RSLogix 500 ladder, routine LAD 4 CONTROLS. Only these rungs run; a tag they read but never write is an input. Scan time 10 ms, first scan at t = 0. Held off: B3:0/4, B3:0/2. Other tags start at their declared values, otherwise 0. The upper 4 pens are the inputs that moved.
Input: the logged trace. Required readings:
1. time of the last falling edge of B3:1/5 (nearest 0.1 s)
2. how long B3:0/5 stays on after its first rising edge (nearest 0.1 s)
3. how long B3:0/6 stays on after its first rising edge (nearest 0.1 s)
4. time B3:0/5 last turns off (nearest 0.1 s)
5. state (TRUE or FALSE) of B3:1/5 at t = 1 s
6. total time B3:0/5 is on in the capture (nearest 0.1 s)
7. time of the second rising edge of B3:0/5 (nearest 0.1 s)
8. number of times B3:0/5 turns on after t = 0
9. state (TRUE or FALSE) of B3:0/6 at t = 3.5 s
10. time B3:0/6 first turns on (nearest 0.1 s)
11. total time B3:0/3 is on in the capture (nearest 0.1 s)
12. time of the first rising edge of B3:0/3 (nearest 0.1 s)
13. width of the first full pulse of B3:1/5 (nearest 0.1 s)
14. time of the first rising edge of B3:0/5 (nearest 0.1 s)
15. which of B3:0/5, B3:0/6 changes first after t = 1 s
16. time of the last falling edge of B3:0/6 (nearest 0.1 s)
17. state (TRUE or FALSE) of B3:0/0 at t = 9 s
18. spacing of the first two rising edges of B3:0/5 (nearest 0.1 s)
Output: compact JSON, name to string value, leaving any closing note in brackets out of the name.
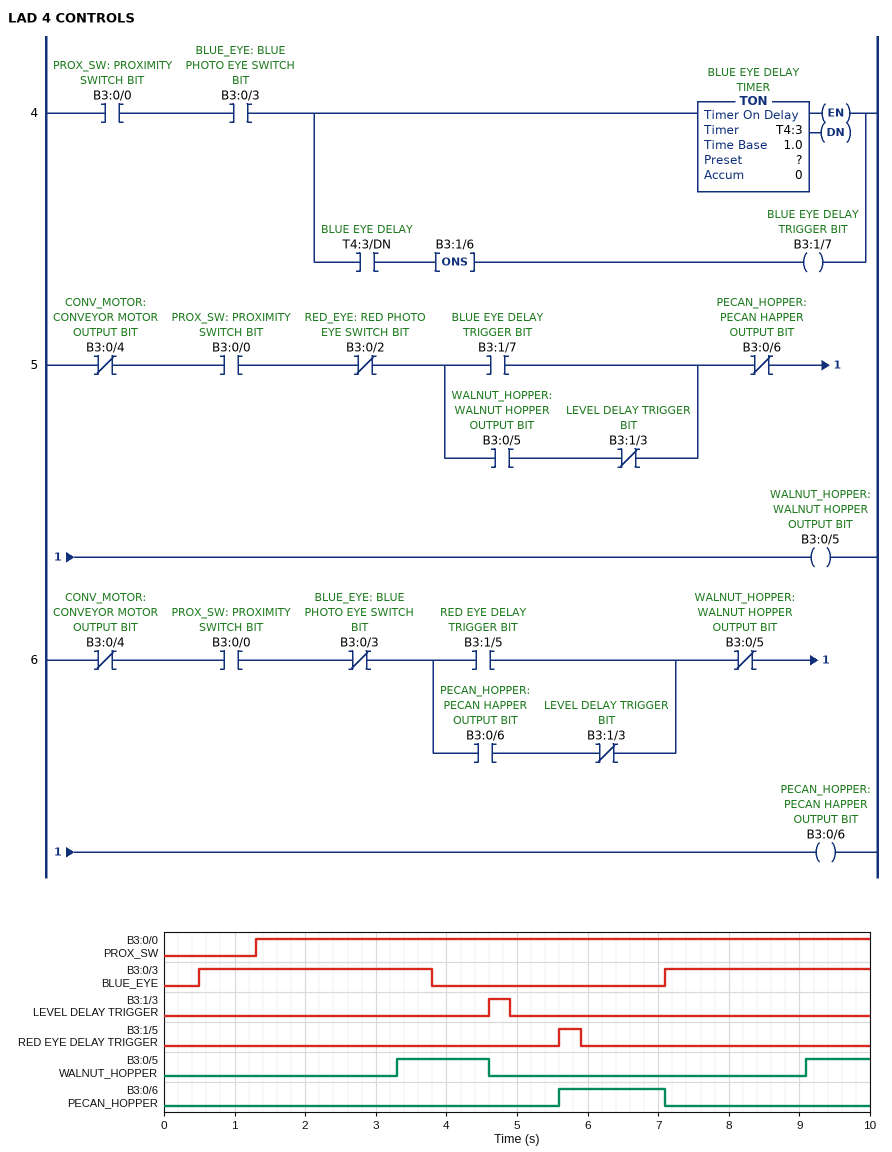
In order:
{"time of the last falling edge of B3:1/5": "5.9 s", "how long B3:0/5 stays on after its first rising edge": "1.3 s", "how long B3:0/6 stays on after its first rising edge": "1.5 s", "time B3:0/5 last turns off": "4.6 s", "state (TRUE or FALSE) of B3:1/5 at t = 1 s": "FALSE", "total time B3:0/5 is on in the capture": "2.2 s", "time of the second rising edge of B3:0/5": "9.1 s", "number of times B3:0/5 turns on after t = 0": "2", "state (TRUE or FALSE) of B3:0/6 at t = 3.5 s": "FALSE", "time B3:0/6 first turns on": "5.6 s", "total time B3:0/3 is on in the capture": "6.2 s", "time of the first rising edge of B3:0/3": "0.5 s", "width of the first full pulse of B3:1/5": "0.3 s", "time of the first rising edge of B3:0/5": "3.3 s", "which of B3:0/5, B3:0/6 changes first after t = 1 s": "B3:0/5", "time of the last falling edge of B3:0/6": "7.1 s", "state (TRUE or FALSE) of B3:0/0 at t = 9 s": "TRUE", "spacing of the first two rising edges of B3:0/5": "5.8 s"}
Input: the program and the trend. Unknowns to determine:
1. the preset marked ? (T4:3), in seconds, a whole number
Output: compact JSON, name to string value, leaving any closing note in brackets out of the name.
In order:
{"the preset marked ? (T4:3), in seconds, a whole number": "2 s"}
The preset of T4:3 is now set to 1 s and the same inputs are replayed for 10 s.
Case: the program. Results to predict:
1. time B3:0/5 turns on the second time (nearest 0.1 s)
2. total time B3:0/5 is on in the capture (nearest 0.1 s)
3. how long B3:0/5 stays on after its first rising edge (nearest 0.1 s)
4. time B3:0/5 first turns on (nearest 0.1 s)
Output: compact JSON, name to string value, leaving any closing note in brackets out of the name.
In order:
{"time B3:0/5 turns on the second time": "8.1 s", "total time B3:0/5 is on in the capture": "4.2 s", "how long B3:0/5 stays on after its first rising edge": "2.3 s", "time B3:0/5 first turns on": "2.3 s"}
